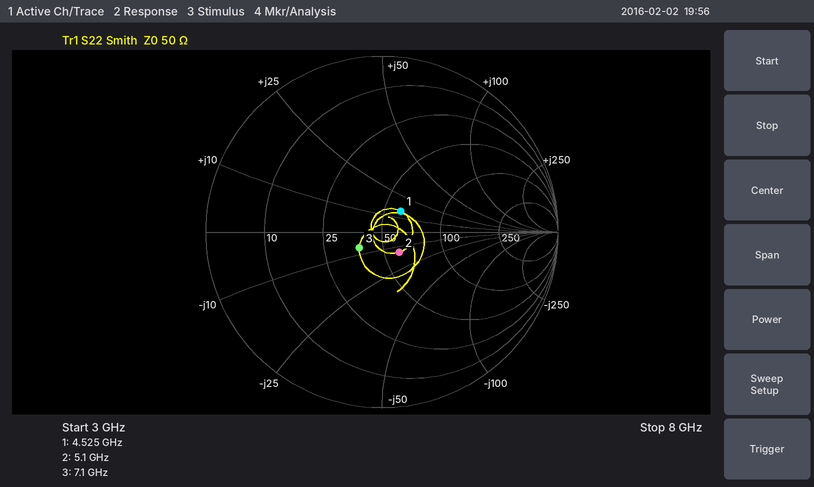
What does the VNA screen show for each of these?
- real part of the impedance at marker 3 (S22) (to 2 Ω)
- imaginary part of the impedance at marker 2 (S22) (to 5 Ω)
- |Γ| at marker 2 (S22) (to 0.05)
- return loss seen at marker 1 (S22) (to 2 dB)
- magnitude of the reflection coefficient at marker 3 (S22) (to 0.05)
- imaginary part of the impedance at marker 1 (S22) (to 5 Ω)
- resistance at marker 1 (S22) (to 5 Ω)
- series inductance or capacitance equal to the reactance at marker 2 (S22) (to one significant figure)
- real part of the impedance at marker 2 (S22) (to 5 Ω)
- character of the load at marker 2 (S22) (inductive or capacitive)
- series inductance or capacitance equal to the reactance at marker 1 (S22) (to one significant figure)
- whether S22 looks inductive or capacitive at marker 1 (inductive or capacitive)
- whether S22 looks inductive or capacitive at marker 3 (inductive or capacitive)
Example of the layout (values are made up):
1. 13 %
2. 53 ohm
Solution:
1. 38 Ω
2. -15 Ω
3. 0.15
4. 16 dB
5. 0.15
6. +15 Ω
7. 60 Ω
8. 2 pF
9. 60 Ω
10. capacitive
11. 500 pH
12. inductive
13. capacitive
